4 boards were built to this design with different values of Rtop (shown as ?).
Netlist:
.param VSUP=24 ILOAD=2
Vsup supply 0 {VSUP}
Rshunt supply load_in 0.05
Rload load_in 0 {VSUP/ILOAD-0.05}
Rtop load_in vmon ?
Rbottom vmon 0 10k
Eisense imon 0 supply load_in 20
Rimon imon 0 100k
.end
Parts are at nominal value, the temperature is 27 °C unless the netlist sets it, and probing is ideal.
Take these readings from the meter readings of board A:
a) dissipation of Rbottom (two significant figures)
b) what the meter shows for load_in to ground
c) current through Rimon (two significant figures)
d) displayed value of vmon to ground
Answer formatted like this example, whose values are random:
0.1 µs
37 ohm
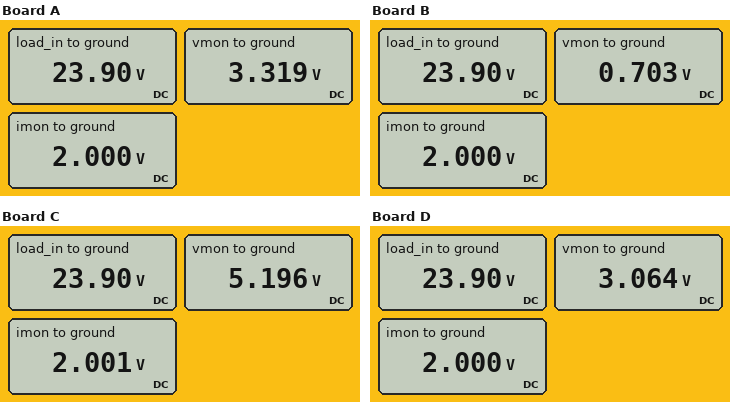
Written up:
1.1 mW
23.90 V
20 µA
3.319 V
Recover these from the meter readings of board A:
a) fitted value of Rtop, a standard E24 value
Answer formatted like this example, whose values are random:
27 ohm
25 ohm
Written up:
62 kΩ
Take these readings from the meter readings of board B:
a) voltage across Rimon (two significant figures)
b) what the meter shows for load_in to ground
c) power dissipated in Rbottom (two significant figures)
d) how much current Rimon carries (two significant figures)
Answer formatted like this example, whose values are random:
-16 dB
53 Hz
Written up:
2.0 V
23.90 V
49 µW
20 µA
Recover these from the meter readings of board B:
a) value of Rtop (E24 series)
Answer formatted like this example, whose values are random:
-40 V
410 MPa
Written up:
330 kΩ
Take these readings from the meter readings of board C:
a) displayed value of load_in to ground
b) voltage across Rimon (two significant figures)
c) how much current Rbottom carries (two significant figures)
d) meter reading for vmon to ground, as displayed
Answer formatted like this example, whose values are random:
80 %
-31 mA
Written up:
23.90 V
2.0 V
520 µA
5.196 V
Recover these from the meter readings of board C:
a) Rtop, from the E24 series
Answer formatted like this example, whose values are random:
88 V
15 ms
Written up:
36 kΩ
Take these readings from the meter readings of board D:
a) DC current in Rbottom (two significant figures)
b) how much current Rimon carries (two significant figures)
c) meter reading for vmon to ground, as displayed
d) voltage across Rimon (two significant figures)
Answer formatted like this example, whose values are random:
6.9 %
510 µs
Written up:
310 µA
20 µA
3.064 V
2.0 V
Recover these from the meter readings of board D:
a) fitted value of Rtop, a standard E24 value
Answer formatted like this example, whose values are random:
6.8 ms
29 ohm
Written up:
68 kΩ
